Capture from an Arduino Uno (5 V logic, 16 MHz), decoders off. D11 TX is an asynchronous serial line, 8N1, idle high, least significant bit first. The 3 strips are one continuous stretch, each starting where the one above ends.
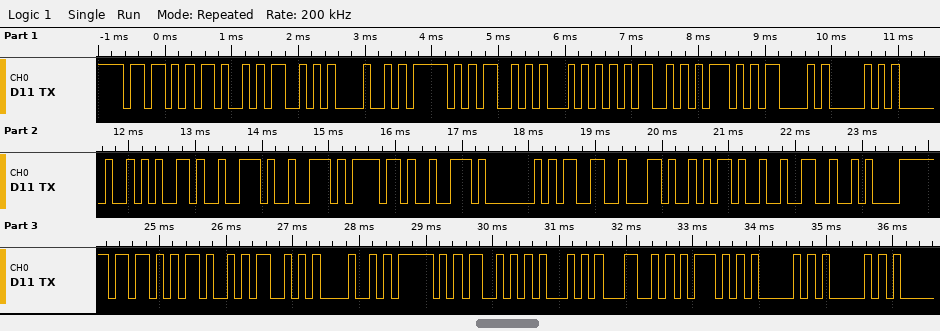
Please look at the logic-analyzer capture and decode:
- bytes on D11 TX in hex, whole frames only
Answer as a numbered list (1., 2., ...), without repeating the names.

1. 5B 4B 53 48 5F 53 54 4D 5D 43 50 20 65 72 72 6F 72 40 33 2C 2D 32 0A 5B 4B 53 48 5F 53 51 4C 5D 41 41
